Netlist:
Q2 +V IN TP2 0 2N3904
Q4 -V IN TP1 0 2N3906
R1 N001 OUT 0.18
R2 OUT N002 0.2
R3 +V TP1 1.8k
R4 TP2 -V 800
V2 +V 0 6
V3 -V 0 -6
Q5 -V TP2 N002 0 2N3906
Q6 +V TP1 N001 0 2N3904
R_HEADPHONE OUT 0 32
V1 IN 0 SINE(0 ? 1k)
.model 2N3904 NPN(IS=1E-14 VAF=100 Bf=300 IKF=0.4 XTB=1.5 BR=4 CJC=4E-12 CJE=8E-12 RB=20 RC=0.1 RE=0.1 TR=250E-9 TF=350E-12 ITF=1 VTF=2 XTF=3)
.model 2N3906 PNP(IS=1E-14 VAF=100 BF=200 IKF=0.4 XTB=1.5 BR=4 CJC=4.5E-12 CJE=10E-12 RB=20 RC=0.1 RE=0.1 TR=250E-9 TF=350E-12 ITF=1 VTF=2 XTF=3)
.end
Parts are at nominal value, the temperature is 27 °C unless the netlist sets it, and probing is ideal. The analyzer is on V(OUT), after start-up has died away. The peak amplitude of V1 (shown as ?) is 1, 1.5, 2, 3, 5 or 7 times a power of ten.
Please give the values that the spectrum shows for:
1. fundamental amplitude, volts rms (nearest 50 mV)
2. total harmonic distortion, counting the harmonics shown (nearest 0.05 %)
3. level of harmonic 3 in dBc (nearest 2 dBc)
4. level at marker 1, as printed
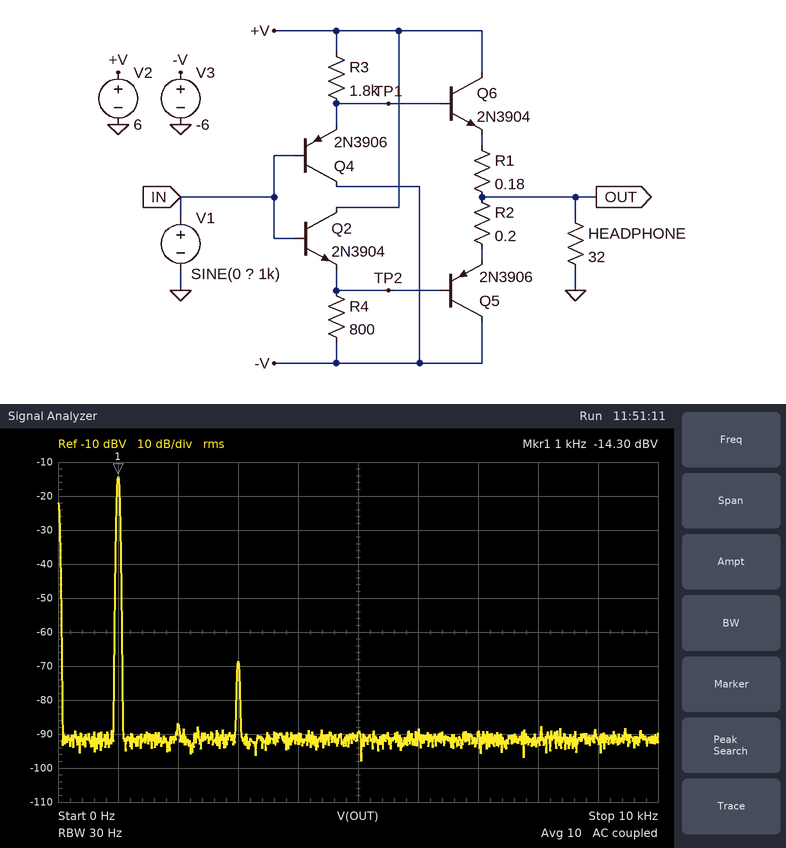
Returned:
200 mV
0.20 %
-54 dBc
-14.30 dBV
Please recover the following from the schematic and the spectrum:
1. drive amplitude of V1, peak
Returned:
300 mV
